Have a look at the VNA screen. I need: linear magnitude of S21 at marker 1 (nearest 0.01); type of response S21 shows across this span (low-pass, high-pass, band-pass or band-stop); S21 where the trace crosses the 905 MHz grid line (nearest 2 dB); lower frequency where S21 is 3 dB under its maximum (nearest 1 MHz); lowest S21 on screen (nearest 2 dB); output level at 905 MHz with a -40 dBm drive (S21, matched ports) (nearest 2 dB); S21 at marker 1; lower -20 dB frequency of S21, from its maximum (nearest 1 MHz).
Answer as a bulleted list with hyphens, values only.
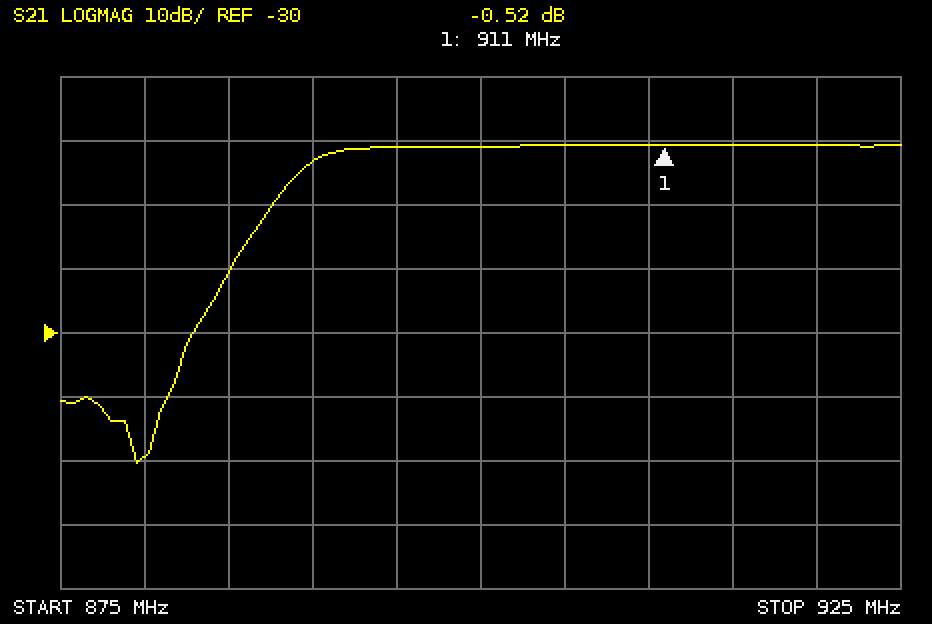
- 0.94
- high-pass
- 0 dB
- 890 MHz
- -50 dB
- -40 dBm
- -0.52 dB
- 885 MHz
